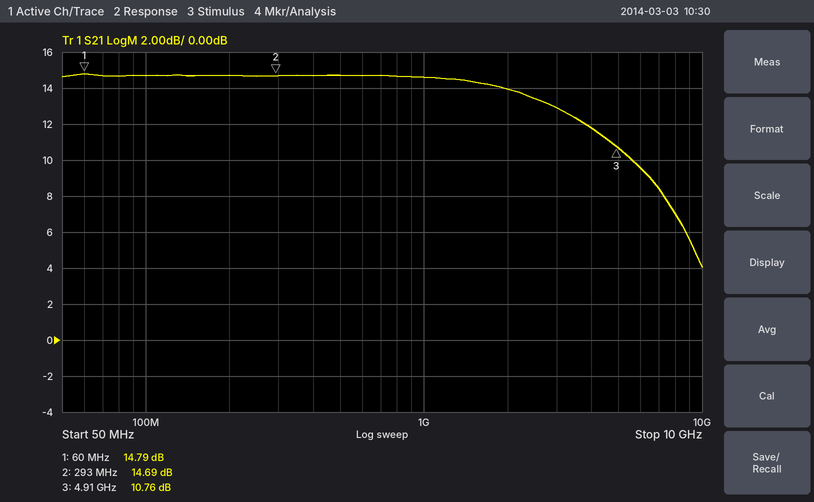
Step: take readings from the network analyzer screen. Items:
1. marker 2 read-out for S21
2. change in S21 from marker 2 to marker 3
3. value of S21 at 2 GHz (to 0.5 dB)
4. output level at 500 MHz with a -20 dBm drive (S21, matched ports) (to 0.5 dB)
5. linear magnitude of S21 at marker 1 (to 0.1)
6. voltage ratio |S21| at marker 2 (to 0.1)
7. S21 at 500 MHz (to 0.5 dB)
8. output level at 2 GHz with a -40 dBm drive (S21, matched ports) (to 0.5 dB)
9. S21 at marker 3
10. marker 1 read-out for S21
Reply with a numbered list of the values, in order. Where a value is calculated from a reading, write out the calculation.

1. 14.69 dB
2. 10.76 − (14.69) = -3.93 dB
3. 14.0 dB
4. -20 dBm + (14.5 dB) = -5.5 dBm
5. 10^(14.79/20) ≈ 5.5
6. 10^(14.69/20) ≈ 5.4
7. 14.5 dB
8. -40 dBm + (14.0 dB) = -26.0 dBm
9. 10.76 dB
10. 14.79 dB
